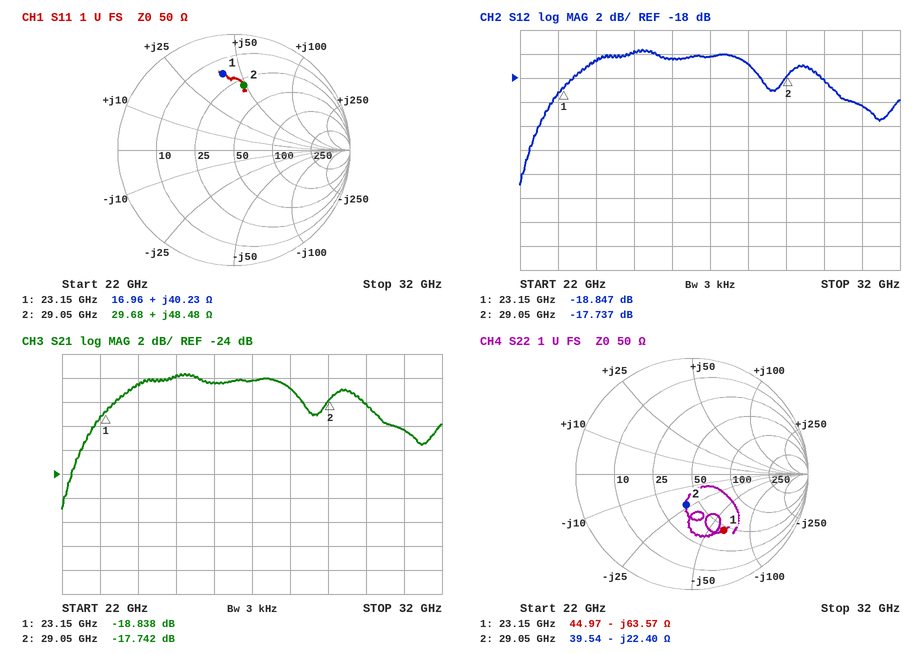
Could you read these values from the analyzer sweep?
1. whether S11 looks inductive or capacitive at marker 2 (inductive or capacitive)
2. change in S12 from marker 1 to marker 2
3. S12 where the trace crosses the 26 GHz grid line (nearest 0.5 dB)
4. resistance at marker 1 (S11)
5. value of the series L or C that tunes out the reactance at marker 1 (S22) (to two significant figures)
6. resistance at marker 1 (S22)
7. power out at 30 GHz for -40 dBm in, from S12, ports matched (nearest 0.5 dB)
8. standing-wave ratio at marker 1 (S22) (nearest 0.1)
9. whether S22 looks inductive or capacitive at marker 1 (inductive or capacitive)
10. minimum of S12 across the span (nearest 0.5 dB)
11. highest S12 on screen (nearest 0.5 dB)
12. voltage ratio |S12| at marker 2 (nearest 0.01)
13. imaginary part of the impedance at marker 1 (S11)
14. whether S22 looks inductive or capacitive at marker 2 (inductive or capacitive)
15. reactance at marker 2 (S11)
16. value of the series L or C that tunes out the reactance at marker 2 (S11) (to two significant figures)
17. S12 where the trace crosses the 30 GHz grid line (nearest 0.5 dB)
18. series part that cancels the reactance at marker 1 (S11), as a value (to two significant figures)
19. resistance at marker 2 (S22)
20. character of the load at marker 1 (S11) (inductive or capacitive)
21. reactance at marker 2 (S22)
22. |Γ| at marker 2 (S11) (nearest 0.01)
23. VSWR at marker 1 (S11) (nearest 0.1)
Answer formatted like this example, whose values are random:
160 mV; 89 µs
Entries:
inductive; 1.110 dB; -16.5 dB; 16.96 Ω; 440 pH; 44.97 Ω; -58.0 dBm; 3.5; capacitive; -27.0 dB; -15.5 dB; 0.13; +40.23 Ω; capacitive; +48.48 Ω; 110 fF; -18.0 dB; 170 fF; 39.54 Ω; inductive; -22.40 Ω; 0.56; 5.0
